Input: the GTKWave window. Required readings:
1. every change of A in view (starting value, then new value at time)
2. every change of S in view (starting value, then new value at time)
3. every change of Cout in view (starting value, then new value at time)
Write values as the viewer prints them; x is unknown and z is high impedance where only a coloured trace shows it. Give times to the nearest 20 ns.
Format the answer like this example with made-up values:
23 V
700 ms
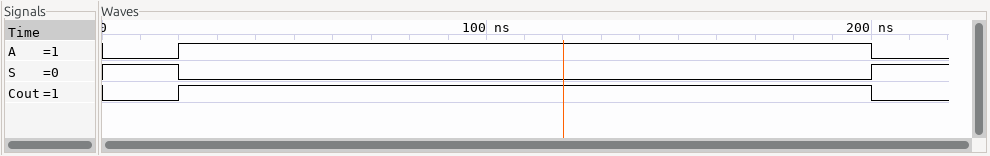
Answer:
0, 1 at 20 ns, 0 at 200 ns
1, 0 at 20 ns, 1 at 200 ns
0, 1 at 20 ns, 0 at 200 ns
